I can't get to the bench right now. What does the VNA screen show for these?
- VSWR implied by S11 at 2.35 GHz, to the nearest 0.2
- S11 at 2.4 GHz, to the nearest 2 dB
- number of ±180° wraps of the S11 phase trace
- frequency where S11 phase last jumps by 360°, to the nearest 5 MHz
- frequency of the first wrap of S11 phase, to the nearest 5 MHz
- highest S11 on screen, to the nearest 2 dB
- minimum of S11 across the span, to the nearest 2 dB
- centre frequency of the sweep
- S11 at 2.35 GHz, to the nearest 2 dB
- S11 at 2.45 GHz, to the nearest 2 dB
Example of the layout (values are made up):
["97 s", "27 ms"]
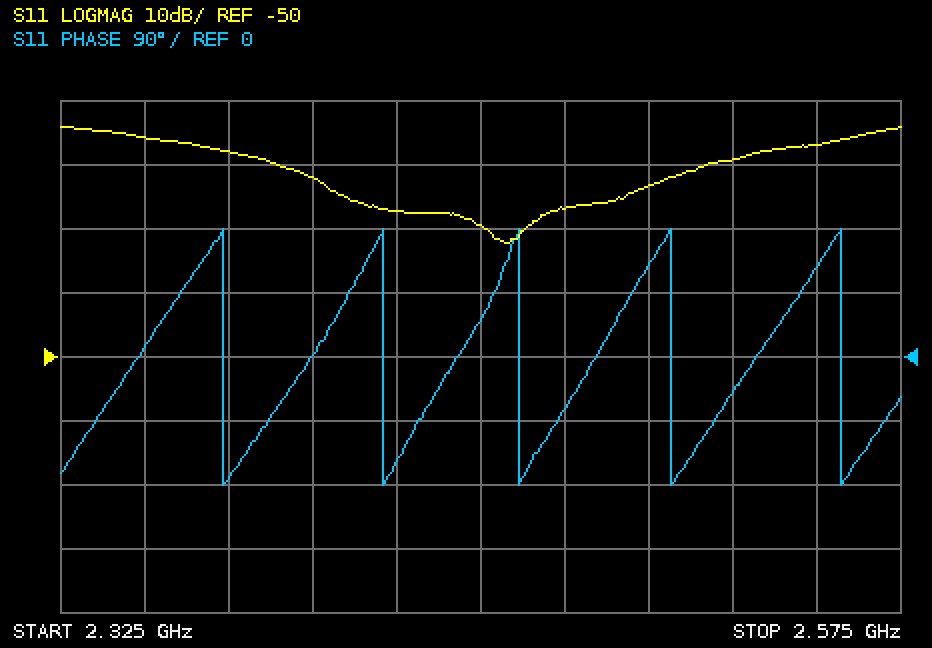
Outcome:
["1.4", "-22 dB", "5", "2.555 GHz", "2.375 GHz", "-14 dB", "-32 dB", "2.45 GHz", "-16 dB", "-30 dB"]
